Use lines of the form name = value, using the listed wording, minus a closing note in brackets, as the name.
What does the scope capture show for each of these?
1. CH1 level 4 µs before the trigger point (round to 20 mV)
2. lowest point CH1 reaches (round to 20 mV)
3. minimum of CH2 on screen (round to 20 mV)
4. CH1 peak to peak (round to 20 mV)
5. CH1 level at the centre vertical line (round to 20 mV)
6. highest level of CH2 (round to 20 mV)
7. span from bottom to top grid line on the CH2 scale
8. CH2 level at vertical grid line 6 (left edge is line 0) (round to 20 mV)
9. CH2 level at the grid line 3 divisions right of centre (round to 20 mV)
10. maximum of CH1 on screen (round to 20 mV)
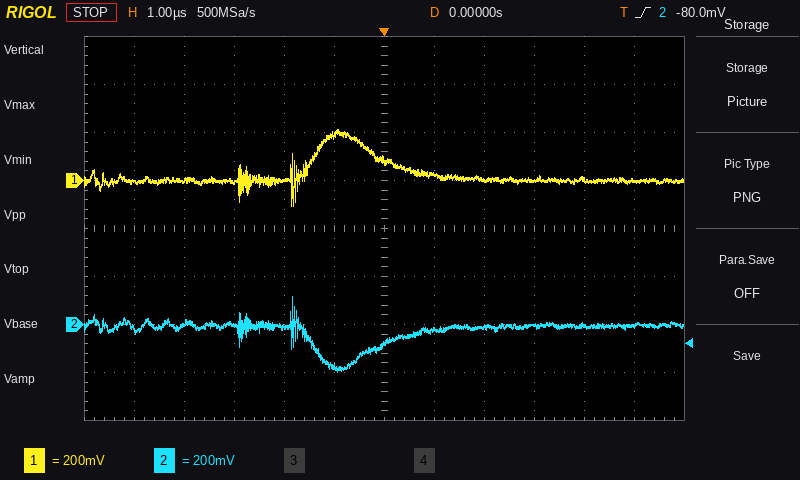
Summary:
CH1 level 4 µs before the trigger point = 0 mV
lowest point CH1 reaches = -100 mV
minimum of CH2 on screen = -200 mV
CH1 peak to peak = 320 mV
CH1 level at the centre vertical line = 80 mV
highest level of CH2 = 120 mV
span from bottom to top grid line on the CH2 scale = 1.6 V
CH2 level at vertical grid line 6 (left edge is line 0) = -80 mV
CH2 level at the grid line 3 divisions right of centre = 0 mV
maximum of CH1 on screen = 220 mV
